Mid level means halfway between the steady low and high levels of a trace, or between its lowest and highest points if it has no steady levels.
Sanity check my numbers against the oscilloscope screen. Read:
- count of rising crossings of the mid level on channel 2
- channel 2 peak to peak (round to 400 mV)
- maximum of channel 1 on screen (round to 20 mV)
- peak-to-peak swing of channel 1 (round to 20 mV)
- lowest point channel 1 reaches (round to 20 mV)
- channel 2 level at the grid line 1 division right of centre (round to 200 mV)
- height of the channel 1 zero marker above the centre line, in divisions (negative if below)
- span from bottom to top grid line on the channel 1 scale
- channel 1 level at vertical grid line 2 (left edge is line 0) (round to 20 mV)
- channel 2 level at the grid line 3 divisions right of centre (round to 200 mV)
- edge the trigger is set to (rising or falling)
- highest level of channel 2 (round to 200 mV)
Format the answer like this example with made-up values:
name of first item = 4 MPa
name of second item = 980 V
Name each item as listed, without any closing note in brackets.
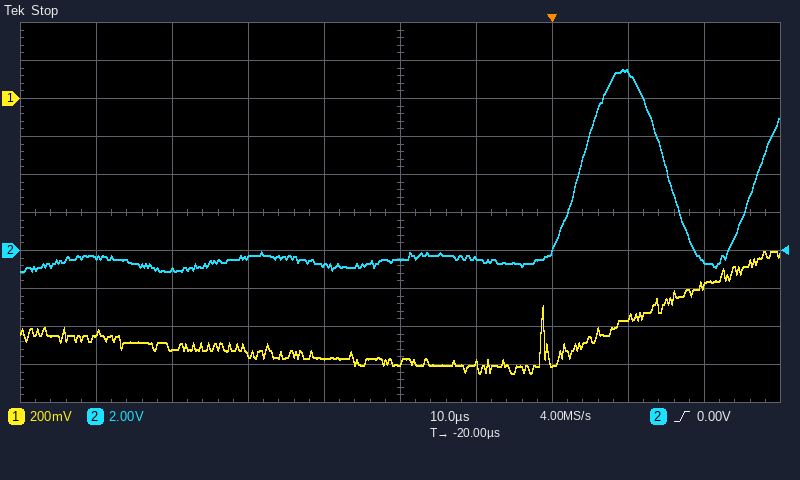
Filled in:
count of rising crossings of the mid level on channel 2 = 2
channel 2 peak to peak = 10.8 V
maximum of channel 1 on screen = -800 mV
peak-to-peak swing of channel 1 = 640 mV
lowest point channel 1 reaches = -1.44 V
channel 2 level at the grid line 1 division right of centre = -400 mV
height of the channel 1 zero marker above the centre line, in divisions = +3.0 div
span from bottom to top grid line on the channel 1 scale = 2 V
channel 1 level at vertical grid line 2 (left edge is line 0) = -1.32 V
channel 2 level at the grid line 3 divisions right of centre = 9.4 V
edge the trigger is set to = rising
highest level of channel 2 = 9.6 V
